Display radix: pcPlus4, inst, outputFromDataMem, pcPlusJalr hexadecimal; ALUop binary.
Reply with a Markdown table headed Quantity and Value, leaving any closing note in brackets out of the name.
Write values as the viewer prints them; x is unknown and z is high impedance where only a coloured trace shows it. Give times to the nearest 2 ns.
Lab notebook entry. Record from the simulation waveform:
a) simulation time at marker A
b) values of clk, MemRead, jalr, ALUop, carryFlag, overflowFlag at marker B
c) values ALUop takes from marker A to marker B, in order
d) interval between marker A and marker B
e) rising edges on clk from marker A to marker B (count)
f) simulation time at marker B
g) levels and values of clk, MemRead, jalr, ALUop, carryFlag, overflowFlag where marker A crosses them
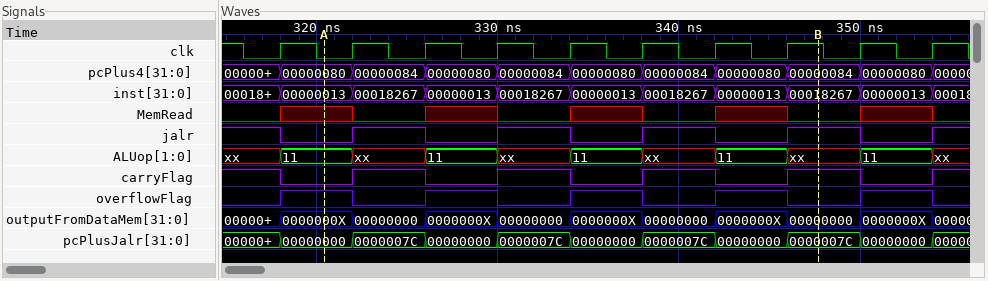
| Quantity | Value |
|---|---|
| simulation time at marker A | 320 ns |
| values of clk, MemRead, jalr, ALUop, carryFlag, overflowFlag at marker B | clk=1, MemRead=0, jalr=1, ALUop=xx, carryFlag=1, overflowFlag=0 |
| values ALUop takes from marker A to marker B, in order | 11, xx, 11, xx, 11, xx, 11, xx |
| interval between marker A and marker B | 28 ns |
| rising edges on clk from marker A to marker B | 7 |
| simulation time at marker B | 348 ns |
| levels and values of clk, MemRead, jalr, ALUop, carryFlag, overflowFlag where marker A crosses them | clk=0, MemRead=x, jalr=0, ALUop=11, carryFlag=0, overflowFlag=1 |
